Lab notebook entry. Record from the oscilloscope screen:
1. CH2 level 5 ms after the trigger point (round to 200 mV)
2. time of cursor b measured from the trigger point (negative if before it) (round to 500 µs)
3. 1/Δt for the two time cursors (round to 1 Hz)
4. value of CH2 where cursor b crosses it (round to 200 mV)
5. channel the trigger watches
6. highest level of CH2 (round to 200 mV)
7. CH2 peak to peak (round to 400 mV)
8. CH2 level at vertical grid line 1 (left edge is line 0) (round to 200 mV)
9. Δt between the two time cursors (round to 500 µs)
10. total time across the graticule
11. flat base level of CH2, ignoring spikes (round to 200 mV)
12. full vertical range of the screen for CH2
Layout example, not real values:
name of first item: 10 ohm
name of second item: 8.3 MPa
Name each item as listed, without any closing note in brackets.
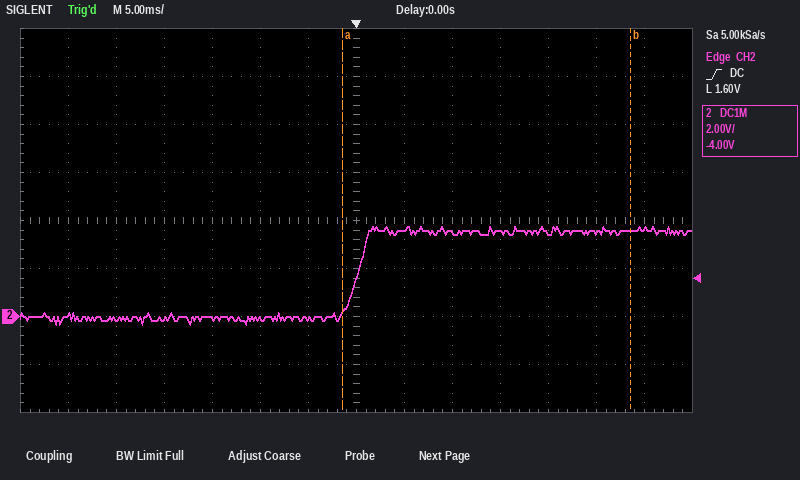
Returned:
CH2 level 5 ms after the trigger point: 3.6 V
time of cursor b measured from the trigger point (negative if before it): +28.5 ms
1/Δt for the two time cursors: 33 Hz
value of CH2 where cursor b crosses it: 3.6 V
channel the trigger watches: CH2
highest level of CH2: 3.8 V
CH2 peak to peak: 4.0 V
CH2 level at vertical grid line 1 (left edge is line 0): 0.0 V
Δt between the two time cursors: 30.0 ms
total time across the graticule: 70 ms
flat base level of CH2, ignoring spikes: 0.0 V
full vertical range of the screen for CH2: 16 V
